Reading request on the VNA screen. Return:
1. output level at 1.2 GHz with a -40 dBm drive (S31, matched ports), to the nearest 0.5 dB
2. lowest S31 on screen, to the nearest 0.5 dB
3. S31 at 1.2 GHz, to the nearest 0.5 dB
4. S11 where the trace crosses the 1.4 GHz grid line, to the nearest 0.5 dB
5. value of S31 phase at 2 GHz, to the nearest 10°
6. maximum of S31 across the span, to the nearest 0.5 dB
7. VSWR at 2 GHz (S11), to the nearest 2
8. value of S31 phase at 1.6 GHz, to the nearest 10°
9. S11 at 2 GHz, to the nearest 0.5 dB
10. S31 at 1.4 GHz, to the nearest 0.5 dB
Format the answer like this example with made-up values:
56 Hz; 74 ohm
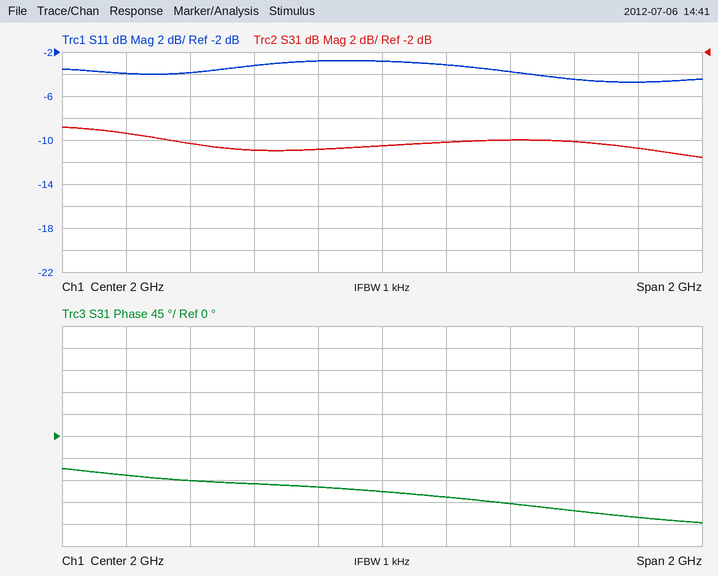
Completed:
-49.5 dBm; -11.5 dB; -9.5 dB; -4.0 dB; -110°; -9.0 dB; 6; -100°; -3.0 dB; -10.5 dB
